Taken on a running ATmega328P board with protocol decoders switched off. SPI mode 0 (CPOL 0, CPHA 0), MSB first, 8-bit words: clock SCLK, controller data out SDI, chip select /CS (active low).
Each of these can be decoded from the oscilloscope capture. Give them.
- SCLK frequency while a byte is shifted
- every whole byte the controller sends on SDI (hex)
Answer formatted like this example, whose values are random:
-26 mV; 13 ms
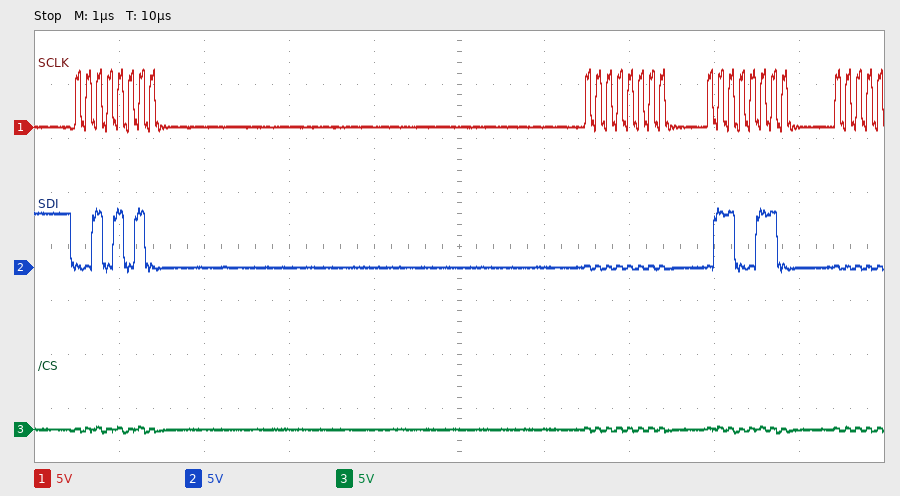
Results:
8 MHz; 2A 00 66
